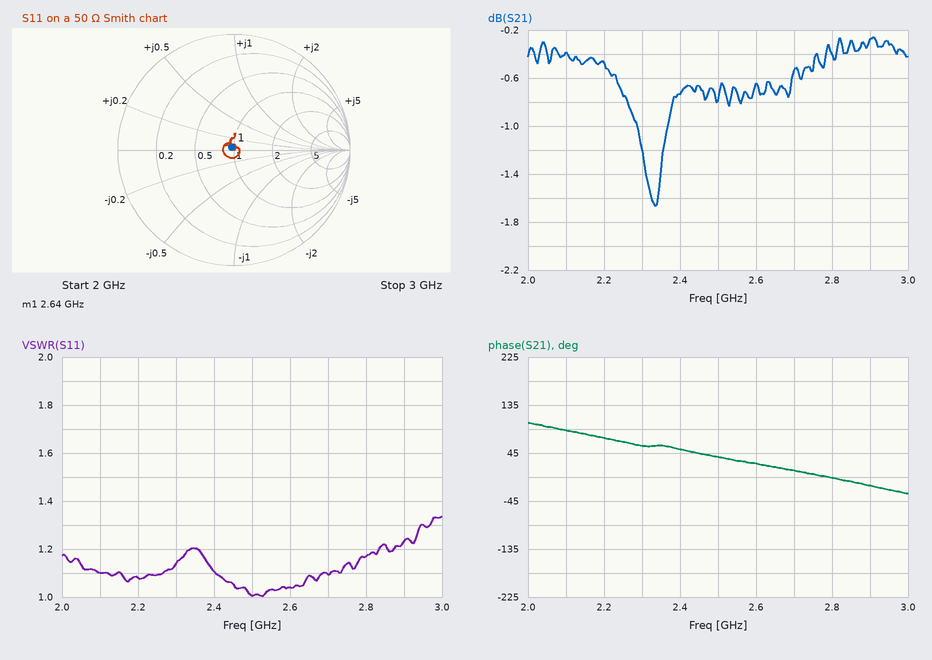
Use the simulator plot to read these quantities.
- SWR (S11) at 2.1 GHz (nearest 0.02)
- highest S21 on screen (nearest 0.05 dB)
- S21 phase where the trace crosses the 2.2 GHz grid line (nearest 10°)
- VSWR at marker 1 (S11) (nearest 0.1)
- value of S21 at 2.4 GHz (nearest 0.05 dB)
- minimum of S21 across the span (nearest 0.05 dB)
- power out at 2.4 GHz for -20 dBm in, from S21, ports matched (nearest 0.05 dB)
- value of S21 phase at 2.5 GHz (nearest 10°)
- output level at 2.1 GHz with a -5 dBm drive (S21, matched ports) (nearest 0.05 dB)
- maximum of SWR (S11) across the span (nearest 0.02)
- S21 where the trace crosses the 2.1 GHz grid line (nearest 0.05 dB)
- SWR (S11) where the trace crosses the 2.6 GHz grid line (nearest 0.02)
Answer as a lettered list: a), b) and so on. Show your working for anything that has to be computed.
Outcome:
a) 1.10
b) -0.25 dB
c) 70°
d) 1.1
e) -0.75 dB
f) -1.65 dB
g) -20 dBm + (-0.75 dB) = -20.75 dBm
h) 40°
i) -5 dBm + (-0.40 dB) = -5.40 dBm
j) 1.34
k) -0.40 dB
l) 1.04
